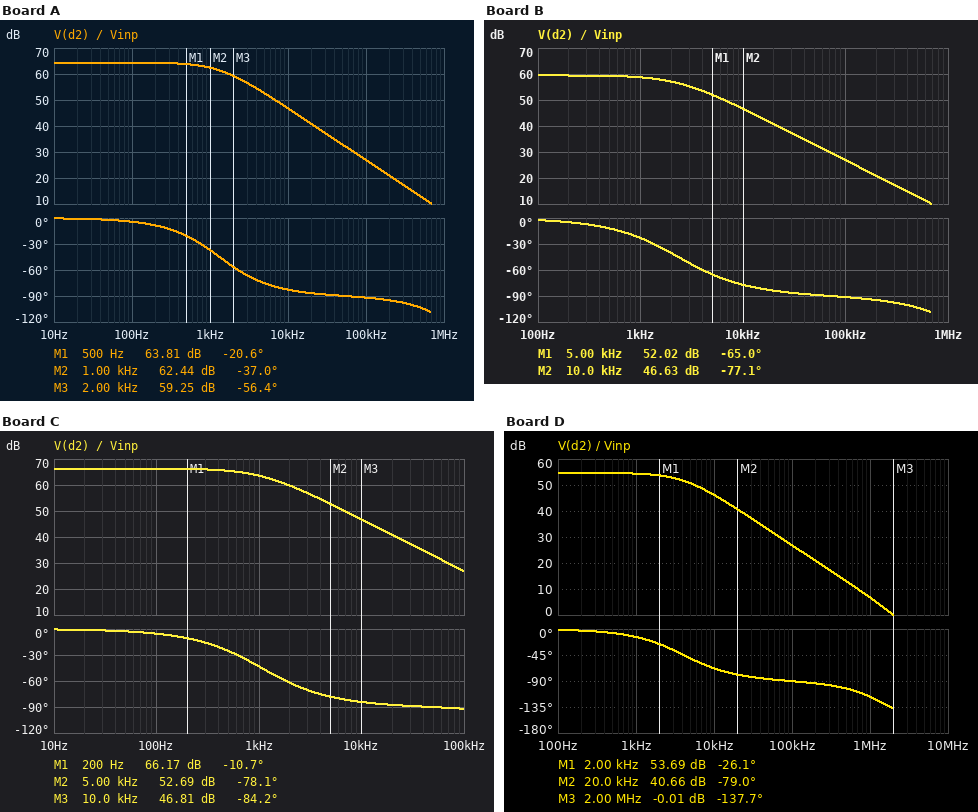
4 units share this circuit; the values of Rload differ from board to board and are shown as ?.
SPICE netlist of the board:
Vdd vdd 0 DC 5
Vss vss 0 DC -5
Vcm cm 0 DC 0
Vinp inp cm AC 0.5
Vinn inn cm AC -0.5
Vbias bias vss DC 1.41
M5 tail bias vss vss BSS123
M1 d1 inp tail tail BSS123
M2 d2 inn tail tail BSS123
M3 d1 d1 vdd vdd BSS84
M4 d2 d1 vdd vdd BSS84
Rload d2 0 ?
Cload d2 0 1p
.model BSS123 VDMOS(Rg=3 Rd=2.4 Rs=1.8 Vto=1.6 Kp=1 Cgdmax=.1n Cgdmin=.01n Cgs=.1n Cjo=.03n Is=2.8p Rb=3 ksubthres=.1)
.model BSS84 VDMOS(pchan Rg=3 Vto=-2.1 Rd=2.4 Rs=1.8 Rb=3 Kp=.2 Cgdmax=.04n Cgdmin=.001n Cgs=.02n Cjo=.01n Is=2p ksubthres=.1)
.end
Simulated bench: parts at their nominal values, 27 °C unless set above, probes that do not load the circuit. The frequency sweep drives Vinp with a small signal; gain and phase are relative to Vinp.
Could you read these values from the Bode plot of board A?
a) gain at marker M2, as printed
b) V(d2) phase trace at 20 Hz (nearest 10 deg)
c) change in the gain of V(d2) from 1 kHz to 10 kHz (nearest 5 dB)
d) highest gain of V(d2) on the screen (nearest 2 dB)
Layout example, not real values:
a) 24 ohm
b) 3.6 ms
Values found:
a) 62.44 dB
b) 0 deg
c) -15 dB
d) 64 dB
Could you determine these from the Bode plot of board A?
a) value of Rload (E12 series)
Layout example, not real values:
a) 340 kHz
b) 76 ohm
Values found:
a) 1.2 MΩ
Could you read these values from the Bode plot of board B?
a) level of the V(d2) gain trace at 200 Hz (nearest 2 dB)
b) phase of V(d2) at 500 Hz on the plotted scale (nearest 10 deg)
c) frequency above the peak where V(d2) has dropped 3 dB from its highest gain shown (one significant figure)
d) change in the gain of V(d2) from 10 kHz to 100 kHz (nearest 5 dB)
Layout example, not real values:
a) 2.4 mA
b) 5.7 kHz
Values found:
a) 60 dB
b) -10 deg
c) 2 kHz
d) -20 dB
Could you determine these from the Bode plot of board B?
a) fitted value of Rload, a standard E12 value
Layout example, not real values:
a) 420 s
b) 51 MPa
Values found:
a) 680 kΩ
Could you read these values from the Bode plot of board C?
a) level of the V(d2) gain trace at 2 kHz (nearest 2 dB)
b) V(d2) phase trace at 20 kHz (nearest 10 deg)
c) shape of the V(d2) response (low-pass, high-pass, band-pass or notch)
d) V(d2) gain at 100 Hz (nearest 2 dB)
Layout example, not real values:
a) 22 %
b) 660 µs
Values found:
a) 60 dB
b) -90 deg
c) low-pass
d) 66 dB
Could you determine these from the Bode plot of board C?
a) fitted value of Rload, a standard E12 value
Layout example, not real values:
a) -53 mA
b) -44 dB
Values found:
a) 1.5 MΩ
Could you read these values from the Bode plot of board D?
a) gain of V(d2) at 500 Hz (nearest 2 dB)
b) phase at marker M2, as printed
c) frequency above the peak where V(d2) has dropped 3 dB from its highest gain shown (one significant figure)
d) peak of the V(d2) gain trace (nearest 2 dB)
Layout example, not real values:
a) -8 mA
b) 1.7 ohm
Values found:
a) 54 dB
b) -79.0 deg
c) 4 kHz
d) 54 dB
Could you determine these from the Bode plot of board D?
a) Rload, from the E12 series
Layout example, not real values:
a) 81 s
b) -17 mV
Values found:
a) 390 kΩ
